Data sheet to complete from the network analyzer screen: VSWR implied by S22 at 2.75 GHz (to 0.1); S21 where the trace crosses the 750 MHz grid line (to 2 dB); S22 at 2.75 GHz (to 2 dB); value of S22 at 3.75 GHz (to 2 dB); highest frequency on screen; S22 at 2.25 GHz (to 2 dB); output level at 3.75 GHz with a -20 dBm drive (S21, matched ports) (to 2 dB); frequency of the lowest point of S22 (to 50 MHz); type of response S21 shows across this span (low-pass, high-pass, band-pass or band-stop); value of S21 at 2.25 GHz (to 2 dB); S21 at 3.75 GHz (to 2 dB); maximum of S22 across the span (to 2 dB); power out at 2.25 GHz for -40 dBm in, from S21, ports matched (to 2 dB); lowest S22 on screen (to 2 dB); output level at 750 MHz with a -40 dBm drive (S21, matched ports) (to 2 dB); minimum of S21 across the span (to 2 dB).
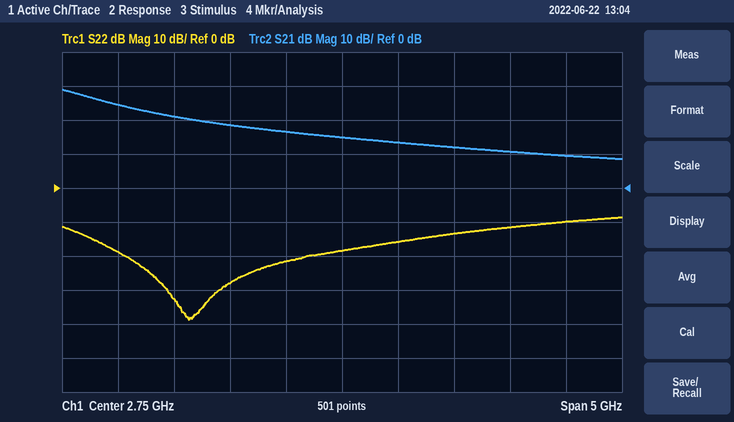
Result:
1.3
24 dB
-18 dB
-14 dB
5.25 GHz
-22 dB
-8 dBm
1.40 GHz
low-pass
16 dB
12 dB
-8 dB
-24 dBm
-38 dB
-16 dBm
8 dB
